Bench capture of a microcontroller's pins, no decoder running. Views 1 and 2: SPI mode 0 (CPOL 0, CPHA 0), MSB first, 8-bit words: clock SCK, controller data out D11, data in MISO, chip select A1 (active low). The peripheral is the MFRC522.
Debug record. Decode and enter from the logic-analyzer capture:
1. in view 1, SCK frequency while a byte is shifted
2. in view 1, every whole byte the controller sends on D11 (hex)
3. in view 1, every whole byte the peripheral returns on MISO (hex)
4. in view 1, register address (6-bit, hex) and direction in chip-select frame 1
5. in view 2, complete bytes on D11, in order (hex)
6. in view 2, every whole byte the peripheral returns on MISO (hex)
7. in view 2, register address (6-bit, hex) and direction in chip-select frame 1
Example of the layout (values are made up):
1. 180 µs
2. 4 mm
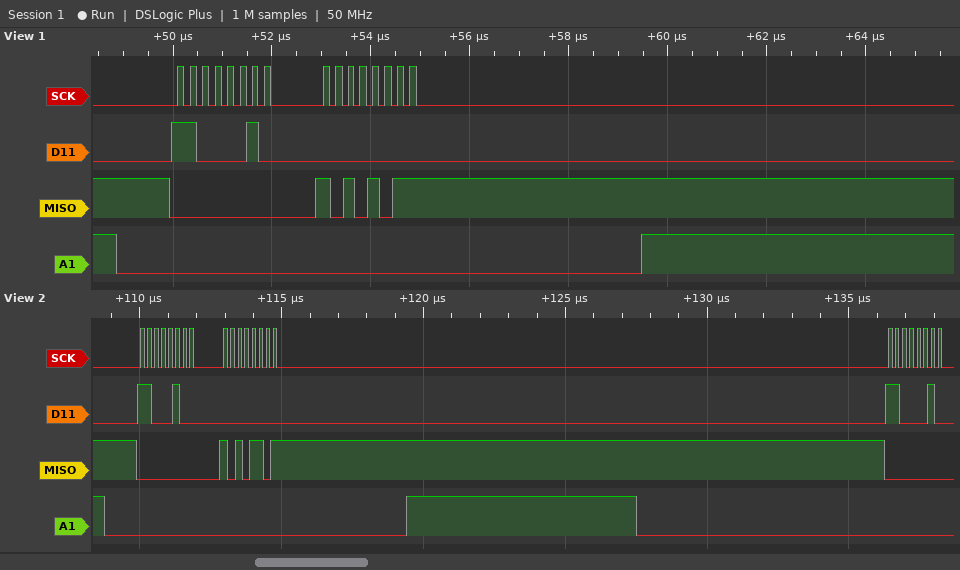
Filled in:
1. 4 MHz
2. C2 00
3. 00 AB
4. 0x21 read
5. C4 00 C2
6. 00 AD 00
7. 0x22 read
